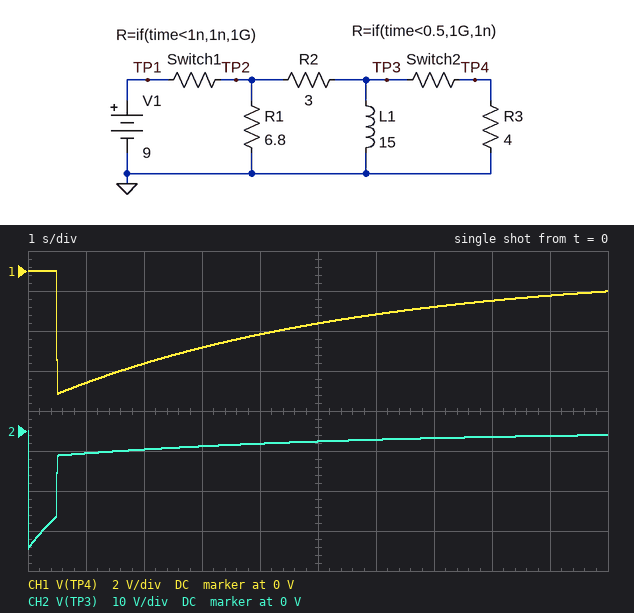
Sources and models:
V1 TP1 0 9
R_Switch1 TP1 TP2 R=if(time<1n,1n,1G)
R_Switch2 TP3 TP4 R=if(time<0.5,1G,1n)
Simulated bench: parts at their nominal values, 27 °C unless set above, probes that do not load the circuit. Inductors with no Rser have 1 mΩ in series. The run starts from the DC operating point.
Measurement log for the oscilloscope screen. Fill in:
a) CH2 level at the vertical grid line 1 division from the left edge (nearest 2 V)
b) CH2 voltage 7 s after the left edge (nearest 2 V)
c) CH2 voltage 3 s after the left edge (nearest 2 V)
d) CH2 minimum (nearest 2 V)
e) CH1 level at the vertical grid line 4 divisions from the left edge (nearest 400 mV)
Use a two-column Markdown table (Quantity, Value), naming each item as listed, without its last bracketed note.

| Quantity | Value |
|---|---|
| CH2 level at the vertical grid line 1 division from the left edge | -6 V |
| CH2 voltage 7 s after the left edge | -2 V |
| CH2 voltage 3 s after the left edge | -4 V |
| CH2 minimum | -30 V |
| CH1 level at the vertical grid line 4 divisions from the left edge | -3.2 V |
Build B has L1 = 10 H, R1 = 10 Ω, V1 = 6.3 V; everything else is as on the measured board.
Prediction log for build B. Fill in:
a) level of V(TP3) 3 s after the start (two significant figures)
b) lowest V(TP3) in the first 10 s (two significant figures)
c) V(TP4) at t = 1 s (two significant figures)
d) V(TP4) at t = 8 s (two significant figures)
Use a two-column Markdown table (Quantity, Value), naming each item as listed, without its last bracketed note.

| Quantity | Value |
|---|---|
| level of V(TP3) 3 s after the start | -1.6 V |
| lowest V(TP3) in the first 10 s | -27 V |
| V(TP4) at t = 1 s | -2.9 V |
| V(TP4) at t = 8 s | -340 mV |
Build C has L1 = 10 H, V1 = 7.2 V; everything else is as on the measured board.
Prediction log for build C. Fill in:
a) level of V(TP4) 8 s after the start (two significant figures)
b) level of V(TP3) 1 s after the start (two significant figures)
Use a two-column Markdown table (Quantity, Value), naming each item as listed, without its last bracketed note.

| Quantity | Value |
|---|---|
| level of V(TP4) 8 s after the start | -500 mV |
| level of V(TP3) 1 s after the start | -3.6 V |
